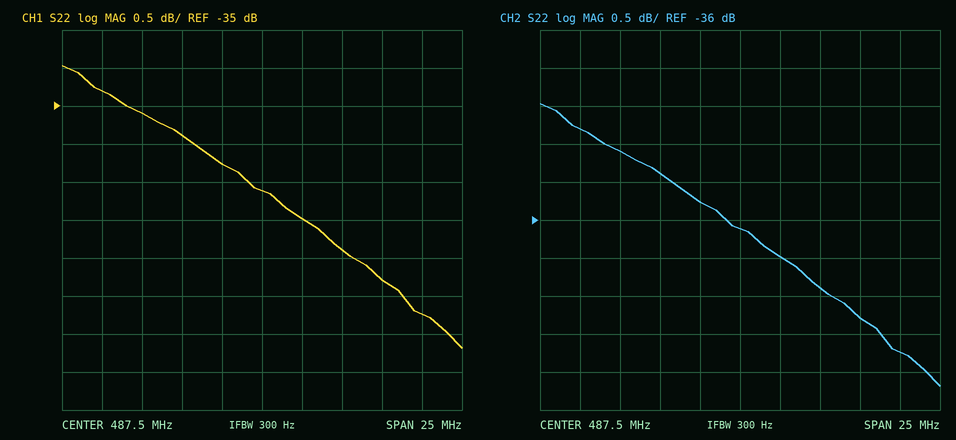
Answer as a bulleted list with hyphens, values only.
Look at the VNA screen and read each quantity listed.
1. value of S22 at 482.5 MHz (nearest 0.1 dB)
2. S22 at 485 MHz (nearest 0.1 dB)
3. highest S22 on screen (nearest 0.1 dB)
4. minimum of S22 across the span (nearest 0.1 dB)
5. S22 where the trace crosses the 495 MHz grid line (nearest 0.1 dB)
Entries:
- -35.4 dB
- -35.8 dB
- -34.5 dB
- -38.2 dB
- -37.3 dB
